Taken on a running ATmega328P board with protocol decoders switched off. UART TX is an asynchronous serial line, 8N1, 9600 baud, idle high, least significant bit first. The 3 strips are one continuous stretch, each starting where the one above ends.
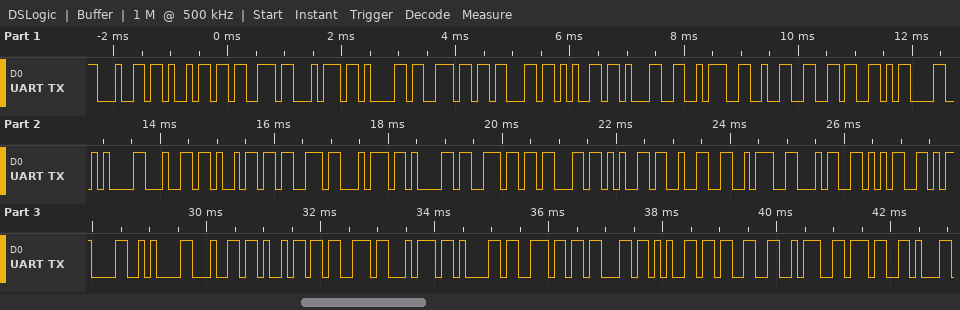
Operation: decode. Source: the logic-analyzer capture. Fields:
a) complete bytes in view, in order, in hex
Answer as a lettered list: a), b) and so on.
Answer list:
a) 0x64 0x69 0x73 0x74 0x61 0x6E 0x63 0x65 0x31 0x3A 0x32 0x36 0x0D 0x0A 0x64 0x69 0x73 0x74 0x61 0x6E 0x63 0x65 0x32 0x3A 0x34 0x35 0x0D 0x0A 0x64 0x69 0x73 0x74 0x61 0x6E 0x63 0x65 0x33 0x3A 0x37
